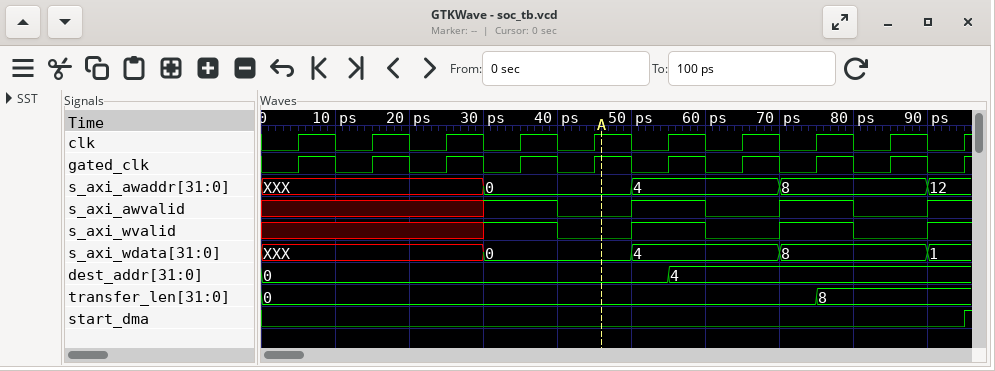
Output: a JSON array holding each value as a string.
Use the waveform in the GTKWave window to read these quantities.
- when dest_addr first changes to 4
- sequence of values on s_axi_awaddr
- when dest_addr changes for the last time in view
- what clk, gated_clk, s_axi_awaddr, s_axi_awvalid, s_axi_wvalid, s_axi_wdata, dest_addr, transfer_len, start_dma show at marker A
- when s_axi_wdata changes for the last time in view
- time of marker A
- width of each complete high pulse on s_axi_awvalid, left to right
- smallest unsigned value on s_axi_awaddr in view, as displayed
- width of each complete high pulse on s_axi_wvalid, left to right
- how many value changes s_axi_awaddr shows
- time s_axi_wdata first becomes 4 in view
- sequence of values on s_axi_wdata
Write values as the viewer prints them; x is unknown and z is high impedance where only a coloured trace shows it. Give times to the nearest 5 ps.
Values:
["55 ps", "XXX, 0, 4, 8, 12", "55 ps", "clk=1, gated_clk=1, s_axi_awaddr=0, s_axi_awvalid=0, s_axi_wvalid=0, s_axi_wdata=0, dest_addr=0, transfer_len=0, start_dma=0", "90 ps", "45 ps", "10 ps, 10 ps", "0", "10 ps, 10 ps", "4", "50 ps", "XXX, 0, 4, 8, 1"]
